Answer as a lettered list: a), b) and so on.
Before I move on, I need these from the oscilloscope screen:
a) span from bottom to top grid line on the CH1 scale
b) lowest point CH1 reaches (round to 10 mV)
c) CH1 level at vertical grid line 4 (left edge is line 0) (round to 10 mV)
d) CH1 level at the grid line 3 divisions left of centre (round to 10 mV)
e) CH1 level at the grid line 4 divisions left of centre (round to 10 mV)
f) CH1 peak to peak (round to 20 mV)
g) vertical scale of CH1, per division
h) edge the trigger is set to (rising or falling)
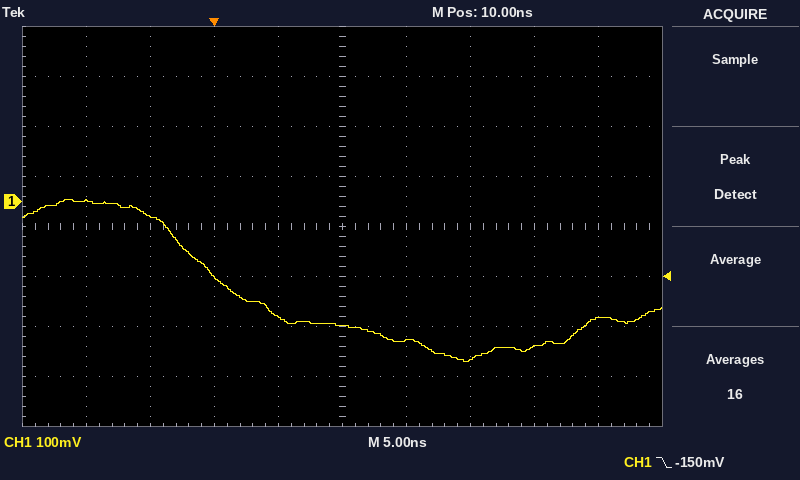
a) 800 mV
b) -320 mV
c) -230 mV
d) -30 mV
e) 0 mV
f) 320 mV
g) 100 mV
h) falling
